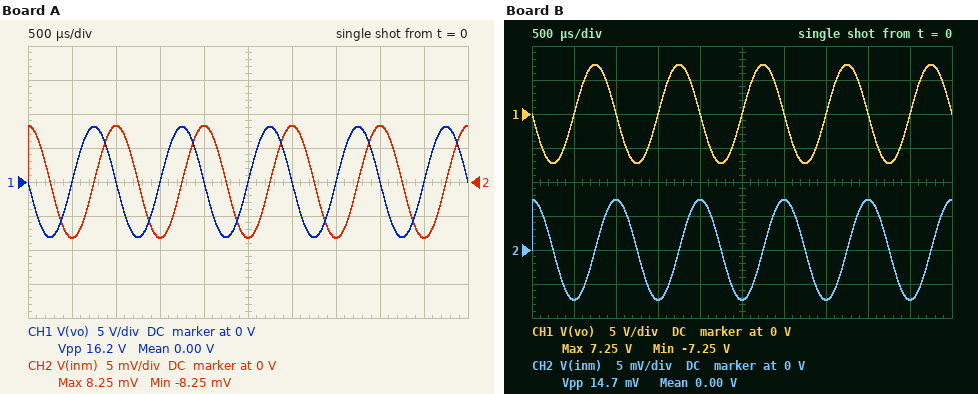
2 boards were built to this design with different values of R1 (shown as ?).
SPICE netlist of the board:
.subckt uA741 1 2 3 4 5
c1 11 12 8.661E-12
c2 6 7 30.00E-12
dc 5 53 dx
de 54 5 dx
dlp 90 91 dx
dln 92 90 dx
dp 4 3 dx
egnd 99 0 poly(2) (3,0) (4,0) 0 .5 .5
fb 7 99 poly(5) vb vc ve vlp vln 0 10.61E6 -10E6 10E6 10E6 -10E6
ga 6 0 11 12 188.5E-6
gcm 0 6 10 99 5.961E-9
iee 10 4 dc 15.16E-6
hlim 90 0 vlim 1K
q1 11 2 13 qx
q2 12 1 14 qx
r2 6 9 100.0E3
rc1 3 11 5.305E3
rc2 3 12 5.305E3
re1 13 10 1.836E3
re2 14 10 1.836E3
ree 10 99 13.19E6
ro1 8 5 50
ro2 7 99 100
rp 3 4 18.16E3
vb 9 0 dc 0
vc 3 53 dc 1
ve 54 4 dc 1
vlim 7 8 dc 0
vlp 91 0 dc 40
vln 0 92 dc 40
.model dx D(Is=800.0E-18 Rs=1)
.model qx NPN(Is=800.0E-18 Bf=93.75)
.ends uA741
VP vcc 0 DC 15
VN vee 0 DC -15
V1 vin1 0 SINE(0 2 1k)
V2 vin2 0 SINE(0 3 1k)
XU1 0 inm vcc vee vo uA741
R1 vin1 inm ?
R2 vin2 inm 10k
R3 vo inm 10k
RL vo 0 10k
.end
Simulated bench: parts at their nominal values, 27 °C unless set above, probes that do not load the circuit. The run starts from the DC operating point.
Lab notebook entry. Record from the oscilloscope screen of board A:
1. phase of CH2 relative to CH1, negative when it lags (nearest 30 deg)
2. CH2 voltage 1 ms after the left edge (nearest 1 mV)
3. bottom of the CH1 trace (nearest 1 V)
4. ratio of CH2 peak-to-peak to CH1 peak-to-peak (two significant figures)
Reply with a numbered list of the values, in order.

1. -90 deg
2. 8 mV
3. -8 V
4. 0.0010
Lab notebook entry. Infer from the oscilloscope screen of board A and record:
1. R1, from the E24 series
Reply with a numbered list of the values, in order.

1. 3.9 kΩ
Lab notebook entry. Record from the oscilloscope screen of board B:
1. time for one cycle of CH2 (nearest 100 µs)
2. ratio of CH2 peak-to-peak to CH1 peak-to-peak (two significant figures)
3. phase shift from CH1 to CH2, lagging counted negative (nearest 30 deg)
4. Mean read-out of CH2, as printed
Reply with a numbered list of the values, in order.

1. 1.0 ms
2. 0.0010
3. -90 deg
4. 0.00 V
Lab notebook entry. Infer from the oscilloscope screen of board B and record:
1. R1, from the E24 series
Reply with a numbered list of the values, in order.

1. 4.7 kΩ
